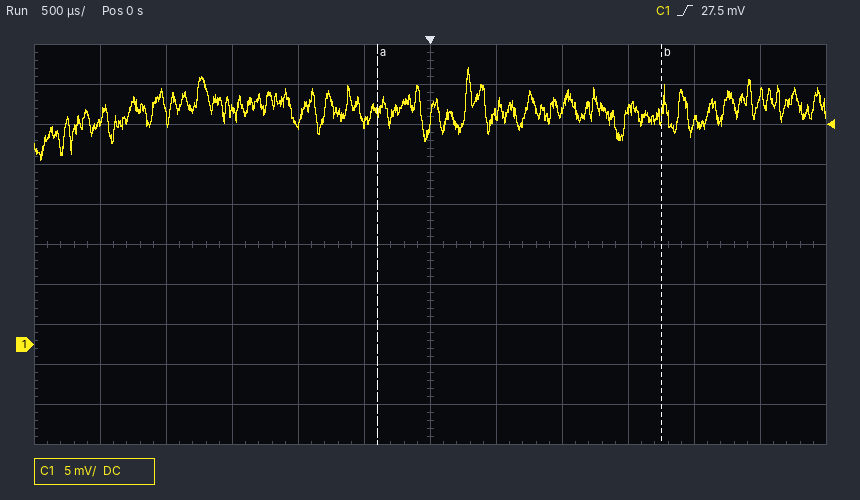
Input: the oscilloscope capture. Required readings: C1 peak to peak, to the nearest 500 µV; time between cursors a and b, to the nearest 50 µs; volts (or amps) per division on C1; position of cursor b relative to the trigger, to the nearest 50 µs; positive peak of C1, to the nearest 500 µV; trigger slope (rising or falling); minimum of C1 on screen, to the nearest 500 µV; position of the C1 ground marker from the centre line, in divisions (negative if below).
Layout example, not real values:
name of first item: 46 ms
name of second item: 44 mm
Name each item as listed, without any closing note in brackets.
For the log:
C1 peak to peak, to the nearest 500 µV: 11.5 mV
time between cursors a and b, to the nearest 50 µs: 2.15 ms
volts (or amps) per division on C1: 5 mV
position of cursor b relative to the trigger, to the nearest 50 µs: +1.75 ms
positive peak of C1, to the nearest 500 µV: 34.5 mV
trigger slope: rising
minimum of C1 on screen, to the nearest 500 µV: 23.0 mV
position of the C1 ground marker from the centre line, in divisions: -2.5 div
